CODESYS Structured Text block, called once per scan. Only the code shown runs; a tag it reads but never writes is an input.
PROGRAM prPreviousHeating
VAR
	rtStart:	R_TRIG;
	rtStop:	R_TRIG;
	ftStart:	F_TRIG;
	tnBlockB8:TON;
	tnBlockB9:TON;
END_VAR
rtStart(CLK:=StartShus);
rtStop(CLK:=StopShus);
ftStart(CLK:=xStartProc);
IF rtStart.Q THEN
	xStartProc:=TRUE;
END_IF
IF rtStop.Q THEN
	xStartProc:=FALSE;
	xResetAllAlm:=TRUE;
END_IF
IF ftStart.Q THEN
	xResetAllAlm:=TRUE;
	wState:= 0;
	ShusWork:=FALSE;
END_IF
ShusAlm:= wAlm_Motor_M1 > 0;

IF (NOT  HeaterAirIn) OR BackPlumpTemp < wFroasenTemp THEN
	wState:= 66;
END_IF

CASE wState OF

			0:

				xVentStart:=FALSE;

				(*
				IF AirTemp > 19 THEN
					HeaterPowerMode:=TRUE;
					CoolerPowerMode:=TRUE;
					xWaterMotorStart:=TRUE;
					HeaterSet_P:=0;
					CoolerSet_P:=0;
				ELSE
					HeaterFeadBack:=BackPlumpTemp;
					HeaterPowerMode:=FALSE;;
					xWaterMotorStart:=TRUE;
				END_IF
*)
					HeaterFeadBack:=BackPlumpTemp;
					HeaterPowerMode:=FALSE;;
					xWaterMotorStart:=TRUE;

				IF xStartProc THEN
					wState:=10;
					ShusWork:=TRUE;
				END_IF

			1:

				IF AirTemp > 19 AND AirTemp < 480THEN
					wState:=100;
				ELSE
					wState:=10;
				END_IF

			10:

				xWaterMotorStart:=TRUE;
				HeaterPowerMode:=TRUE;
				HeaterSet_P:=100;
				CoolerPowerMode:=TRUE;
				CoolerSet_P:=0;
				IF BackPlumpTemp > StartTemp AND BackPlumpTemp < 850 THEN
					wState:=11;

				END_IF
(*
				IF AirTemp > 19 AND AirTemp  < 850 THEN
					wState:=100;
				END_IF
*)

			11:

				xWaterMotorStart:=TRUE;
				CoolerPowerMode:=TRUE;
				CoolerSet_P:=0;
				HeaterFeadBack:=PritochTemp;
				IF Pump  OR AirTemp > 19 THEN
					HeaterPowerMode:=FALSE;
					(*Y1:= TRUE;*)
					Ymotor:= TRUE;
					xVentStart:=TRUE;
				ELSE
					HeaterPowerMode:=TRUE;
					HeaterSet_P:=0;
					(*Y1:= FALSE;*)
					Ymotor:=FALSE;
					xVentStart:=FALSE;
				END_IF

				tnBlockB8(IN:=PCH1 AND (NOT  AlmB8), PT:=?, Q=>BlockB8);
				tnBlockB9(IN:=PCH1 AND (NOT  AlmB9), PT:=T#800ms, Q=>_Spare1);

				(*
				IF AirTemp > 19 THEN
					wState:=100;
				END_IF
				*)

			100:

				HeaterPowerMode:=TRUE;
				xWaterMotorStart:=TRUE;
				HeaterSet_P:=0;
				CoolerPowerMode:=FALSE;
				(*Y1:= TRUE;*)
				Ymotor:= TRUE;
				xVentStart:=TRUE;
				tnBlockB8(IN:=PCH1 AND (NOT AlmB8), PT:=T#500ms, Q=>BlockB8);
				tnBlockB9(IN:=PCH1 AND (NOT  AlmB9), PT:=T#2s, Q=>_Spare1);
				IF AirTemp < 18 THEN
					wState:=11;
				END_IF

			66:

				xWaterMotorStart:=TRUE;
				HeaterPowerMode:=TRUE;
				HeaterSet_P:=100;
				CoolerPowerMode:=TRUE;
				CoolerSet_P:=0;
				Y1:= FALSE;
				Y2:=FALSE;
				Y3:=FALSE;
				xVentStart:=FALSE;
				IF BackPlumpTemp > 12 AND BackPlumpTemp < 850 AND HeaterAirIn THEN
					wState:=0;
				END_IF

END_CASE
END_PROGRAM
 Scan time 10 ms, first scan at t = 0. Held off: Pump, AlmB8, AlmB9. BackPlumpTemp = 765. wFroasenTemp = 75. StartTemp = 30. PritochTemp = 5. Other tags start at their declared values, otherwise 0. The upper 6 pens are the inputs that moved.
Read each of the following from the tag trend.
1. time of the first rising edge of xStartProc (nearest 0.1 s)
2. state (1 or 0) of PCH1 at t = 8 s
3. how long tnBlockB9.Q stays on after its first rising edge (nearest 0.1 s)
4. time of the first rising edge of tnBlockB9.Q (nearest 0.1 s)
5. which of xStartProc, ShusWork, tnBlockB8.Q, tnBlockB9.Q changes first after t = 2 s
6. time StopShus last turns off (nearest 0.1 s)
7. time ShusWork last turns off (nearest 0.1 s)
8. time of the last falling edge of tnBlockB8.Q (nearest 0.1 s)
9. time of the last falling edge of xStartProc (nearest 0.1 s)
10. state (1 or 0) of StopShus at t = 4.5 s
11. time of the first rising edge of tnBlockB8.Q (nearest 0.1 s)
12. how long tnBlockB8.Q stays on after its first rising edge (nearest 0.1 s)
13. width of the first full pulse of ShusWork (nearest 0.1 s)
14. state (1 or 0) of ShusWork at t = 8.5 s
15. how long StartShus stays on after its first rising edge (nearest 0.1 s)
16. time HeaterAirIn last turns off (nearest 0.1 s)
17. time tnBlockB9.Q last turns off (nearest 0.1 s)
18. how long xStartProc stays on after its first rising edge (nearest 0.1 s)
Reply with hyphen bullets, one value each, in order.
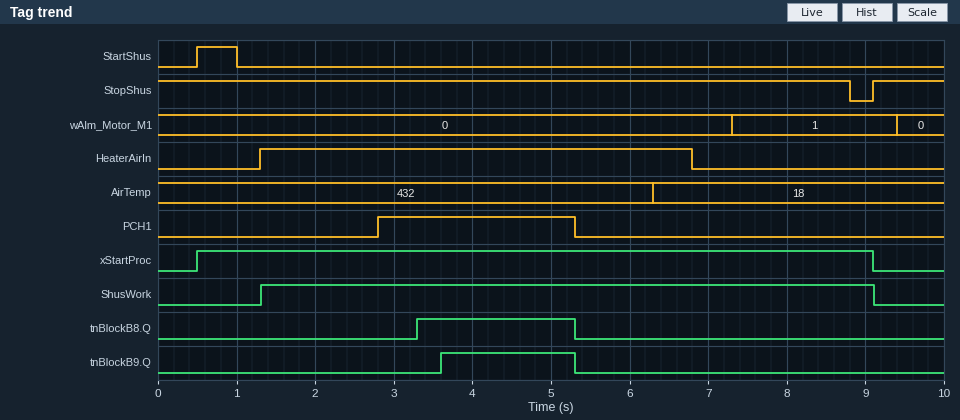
- 0.5 s
- 0
- 1.7 s
- 3.6 s
- tnBlockB8.Q
- 8.8 s
- 9.1 s
- 5.3 s
- 9.1 s
- 1
- 3.3 s
- 2.0 s
- 7.8 s
- 1
- 0.5 s
- 6.8 s
- 5.3 s
- 8.6 s
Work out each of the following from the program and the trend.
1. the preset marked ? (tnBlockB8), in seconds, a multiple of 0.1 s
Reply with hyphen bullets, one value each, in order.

- 0.5 s
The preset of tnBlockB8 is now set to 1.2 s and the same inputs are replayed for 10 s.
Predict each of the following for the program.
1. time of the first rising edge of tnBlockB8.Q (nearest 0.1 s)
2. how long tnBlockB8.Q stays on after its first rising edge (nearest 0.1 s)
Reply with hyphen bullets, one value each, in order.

- 4.0 s
- 1.3 s
